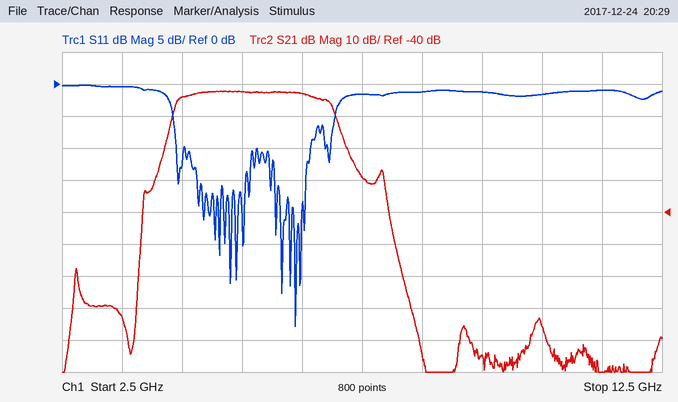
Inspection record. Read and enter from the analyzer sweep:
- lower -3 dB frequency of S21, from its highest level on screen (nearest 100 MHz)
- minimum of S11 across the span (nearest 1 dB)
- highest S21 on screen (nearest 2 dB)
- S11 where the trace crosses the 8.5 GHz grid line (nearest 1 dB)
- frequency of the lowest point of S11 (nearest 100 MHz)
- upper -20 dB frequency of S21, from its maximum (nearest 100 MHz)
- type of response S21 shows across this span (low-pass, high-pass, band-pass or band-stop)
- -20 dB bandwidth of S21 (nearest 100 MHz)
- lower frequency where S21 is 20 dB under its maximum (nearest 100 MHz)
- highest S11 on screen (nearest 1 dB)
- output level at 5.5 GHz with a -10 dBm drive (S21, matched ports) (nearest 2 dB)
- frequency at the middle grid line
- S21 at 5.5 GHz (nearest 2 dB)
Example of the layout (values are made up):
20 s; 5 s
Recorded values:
4.4 GHz; -38 dB; -2 dB; -1 dB; 6.4 GHz; 7.3 GHz; band-pass; 3.1 GHz; 4.2 GHz; 0 dB; -12 dBm; 7.5 GHz; -2 dB
